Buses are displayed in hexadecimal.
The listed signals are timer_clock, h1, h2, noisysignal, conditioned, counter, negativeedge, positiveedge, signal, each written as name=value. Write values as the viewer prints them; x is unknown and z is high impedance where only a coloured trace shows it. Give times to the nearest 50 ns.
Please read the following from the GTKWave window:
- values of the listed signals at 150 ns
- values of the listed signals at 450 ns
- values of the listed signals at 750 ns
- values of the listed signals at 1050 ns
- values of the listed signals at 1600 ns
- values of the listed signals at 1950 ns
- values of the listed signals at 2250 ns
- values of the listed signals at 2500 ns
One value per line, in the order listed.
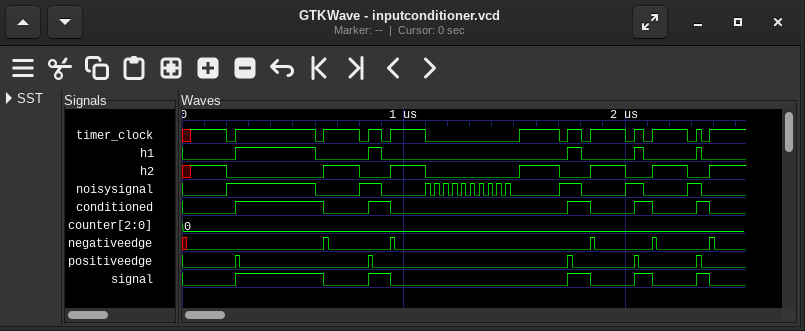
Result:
timer_clock=1, h1=0, h2=1, noisysignal=0, conditioned=0, counter=0, negativeedge=0, positiveedge=0, signal=0
timer_clock=1, h1=1, h2=0, noisysignal=1, conditioned=1, counter=0, negativeedge=0, positiveedge=0, signal=1
timer_clock=1, h1=0, h2=1, noisysignal=0, conditioned=0, counter=0, negativeedge=0, positiveedge=0, signal=0
timer_clock=1, h1=0, h2=1, noisysignal=0, conditioned=0, counter=0, negativeedge=0, positiveedge=0, signal=0
timer_clock=1, h1=0, h2=1, noisysignal=0, conditioned=0, counter=0, negativeedge=0, positiveedge=0, signal=0
timer_clock=1, h1=0, h2=1, noisysignal=0, conditioned=0, counter=0, negativeedge=0, positiveedge=0, signal=0
timer_clock=1, h1=0, h2=1, noisysignal=0, conditioned=0, counter=0, negativeedge=0, positiveedge=0, signal=0
timer_clock=1, h1=0, h2=1, noisysignal=0, conditioned=0, counter=0, negativeedge=0, positiveedge=0, signal=0
